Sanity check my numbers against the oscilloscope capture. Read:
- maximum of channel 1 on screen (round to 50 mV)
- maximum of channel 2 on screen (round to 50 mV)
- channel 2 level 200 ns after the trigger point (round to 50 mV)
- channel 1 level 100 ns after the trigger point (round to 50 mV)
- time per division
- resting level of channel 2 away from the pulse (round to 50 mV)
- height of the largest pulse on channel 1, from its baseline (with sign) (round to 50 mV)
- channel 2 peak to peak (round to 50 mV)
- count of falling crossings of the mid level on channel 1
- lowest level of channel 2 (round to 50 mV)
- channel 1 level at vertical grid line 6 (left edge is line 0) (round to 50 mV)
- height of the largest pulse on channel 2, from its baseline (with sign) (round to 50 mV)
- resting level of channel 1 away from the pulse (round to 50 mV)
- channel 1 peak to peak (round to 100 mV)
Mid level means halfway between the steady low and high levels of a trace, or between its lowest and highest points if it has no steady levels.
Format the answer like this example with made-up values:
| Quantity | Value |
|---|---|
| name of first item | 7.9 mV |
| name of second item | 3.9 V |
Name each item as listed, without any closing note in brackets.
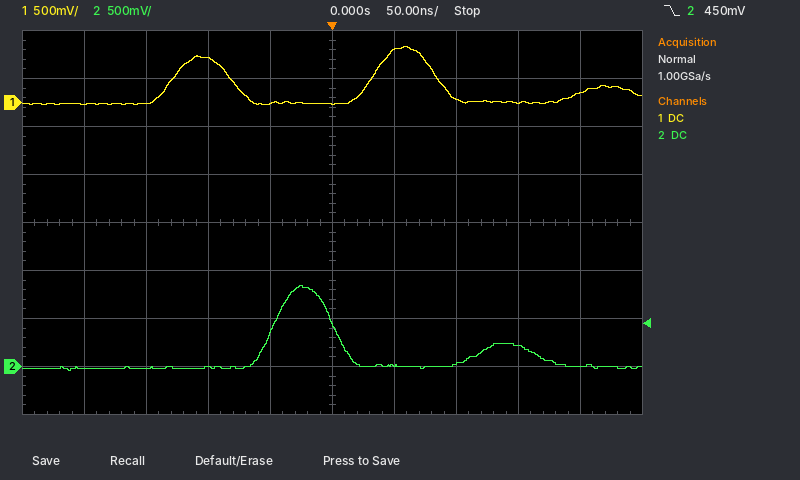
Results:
| Quantity | Value |
|---|---|
| maximum of channel 1 on screen | 600 mV |
| maximum of channel 2 on screen | 850 mV |
| channel 2 level 200 ns after the trigger point | 0 mV |
| channel 1 level 100 ns after the trigger point | 50 mV |
| time per division | 50 ns |
| resting level of channel 2 away from the pulse | 0 mV |
| height of the largest pulse on channel 1, from its baseline (with sign) | +600 mV |
| channel 2 peak to peak | 900 mV |
| count of falling crossings of the mid level on channel 1 | 2 |
| lowest level of channel 2 | -50 mV |
| channel 1 level at vertical grid line 6 (left edge is line 0) | 550 mV |
| height of the largest pulse on channel 2, from its baseline (with sign) | +850 mV |
| resting level of channel 1 away from the pulse | 0 mV |
| channel 1 peak to peak | 600 mV |
